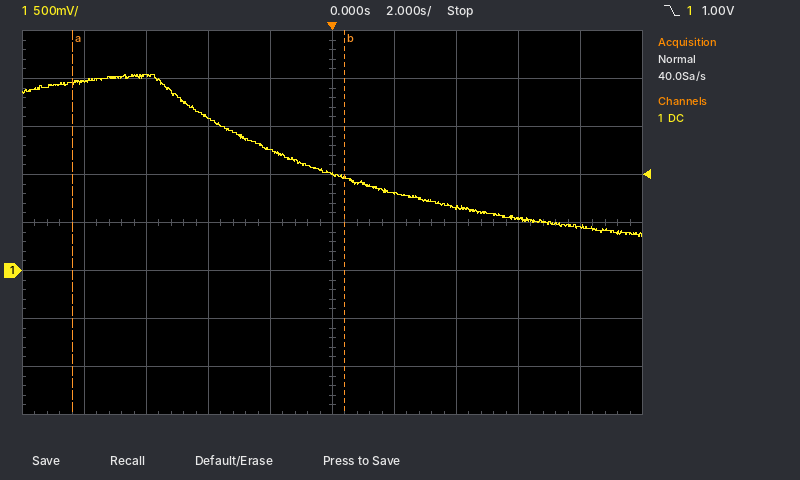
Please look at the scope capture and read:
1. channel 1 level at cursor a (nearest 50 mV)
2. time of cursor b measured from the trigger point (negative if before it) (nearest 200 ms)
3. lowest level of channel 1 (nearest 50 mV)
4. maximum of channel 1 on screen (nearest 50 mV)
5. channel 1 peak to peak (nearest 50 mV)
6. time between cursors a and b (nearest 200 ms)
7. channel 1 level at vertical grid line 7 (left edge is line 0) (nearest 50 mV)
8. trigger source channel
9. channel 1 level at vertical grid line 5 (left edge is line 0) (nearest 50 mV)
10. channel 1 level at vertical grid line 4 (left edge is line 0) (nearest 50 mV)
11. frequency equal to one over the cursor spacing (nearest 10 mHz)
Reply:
1.95 V
+400 ms
350 mV
2.05 V
1.70 V
8.8 s
650 mV
channel 1
1.00 V
1.25 V
110 mHz
